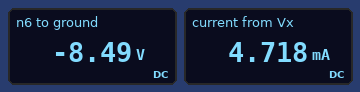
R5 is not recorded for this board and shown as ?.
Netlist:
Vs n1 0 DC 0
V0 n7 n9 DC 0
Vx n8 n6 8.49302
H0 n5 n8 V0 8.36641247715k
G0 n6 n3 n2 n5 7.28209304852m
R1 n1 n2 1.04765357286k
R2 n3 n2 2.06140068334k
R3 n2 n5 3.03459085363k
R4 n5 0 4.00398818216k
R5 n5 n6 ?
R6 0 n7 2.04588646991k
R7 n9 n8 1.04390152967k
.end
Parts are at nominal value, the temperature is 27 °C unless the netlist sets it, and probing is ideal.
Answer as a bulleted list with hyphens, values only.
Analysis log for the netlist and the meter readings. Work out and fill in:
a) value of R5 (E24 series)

- 1.8 kΩ
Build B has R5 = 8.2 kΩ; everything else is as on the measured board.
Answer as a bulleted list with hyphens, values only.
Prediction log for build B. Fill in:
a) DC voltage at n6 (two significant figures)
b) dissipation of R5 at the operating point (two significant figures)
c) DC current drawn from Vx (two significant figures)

- -8.5 V
- 8.8 mW
- 1.0 mA
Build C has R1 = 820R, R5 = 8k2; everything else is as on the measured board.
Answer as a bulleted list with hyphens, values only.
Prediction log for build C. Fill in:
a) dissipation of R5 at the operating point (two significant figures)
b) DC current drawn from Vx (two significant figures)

- 8.8 mW
- 1.0 mA
